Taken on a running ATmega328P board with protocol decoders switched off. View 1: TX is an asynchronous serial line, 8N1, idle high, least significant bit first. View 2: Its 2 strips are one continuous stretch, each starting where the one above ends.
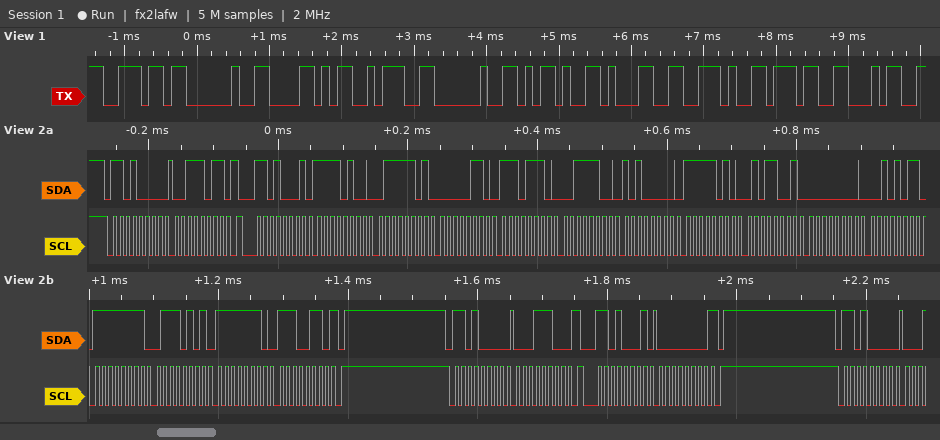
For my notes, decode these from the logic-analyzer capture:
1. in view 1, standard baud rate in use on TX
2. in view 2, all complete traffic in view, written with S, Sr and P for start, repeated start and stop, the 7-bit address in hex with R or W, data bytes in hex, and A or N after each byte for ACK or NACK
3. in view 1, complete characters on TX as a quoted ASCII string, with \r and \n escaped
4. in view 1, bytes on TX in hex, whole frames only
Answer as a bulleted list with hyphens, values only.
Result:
- 9600 baud
- S 68W A 3B A Sr 68R A F4 A 7D A 06 A EE A 3C A A0 A FA A 59 A 00 A 2B A FF A 75 A FE A E6 N P S 68W A 1C A Sr 68R A 00 N P S 68W A
- "n X: -1.74"
- 6E 20 58 3A 20 2D 31 2E 37 34
